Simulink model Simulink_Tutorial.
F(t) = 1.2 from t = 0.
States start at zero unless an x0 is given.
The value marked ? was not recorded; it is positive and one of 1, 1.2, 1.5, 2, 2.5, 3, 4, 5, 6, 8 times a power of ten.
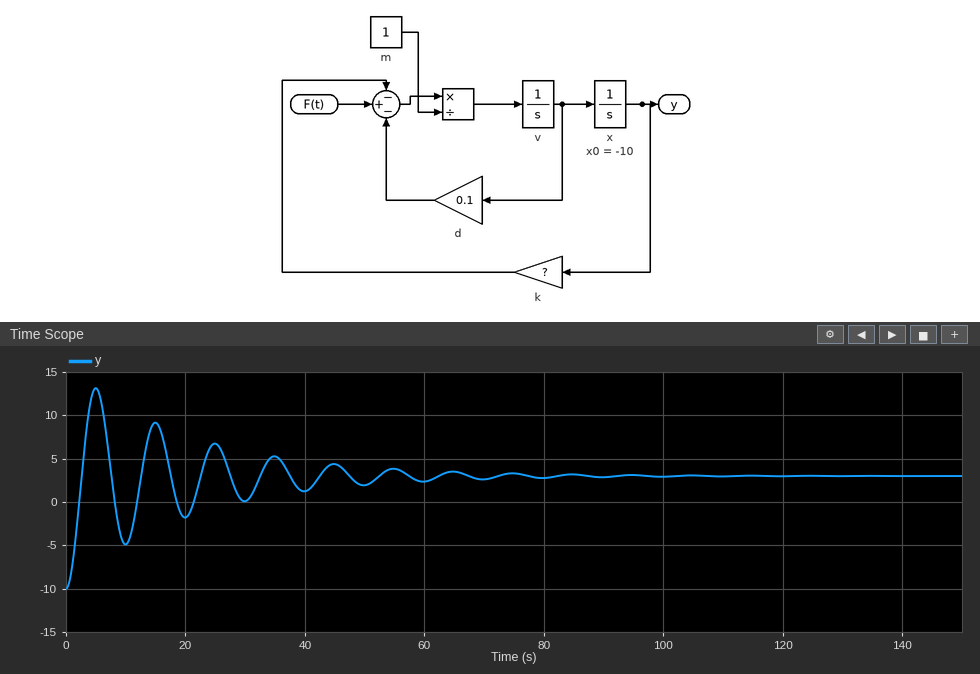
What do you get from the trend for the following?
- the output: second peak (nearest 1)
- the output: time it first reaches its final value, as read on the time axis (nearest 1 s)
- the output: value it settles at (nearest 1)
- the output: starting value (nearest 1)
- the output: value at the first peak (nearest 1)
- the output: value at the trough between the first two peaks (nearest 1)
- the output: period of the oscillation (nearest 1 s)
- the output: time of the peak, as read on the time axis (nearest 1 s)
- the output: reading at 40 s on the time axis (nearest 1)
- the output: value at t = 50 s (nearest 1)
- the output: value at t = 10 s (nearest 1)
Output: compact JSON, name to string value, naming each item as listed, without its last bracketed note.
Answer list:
{"the output: second peak": "9", "the output: time it first reaches its final value, as read on the time axis": "3 s", "the output: value it settles at": "3", "the output: starting value": "-10", "the output: value at the first peak": "13", "the output: value at the trough between the first two peaks": "-5", "the output: period of the oscillation": "10 s", "the output: time of the peak, as read on the time axis": "5 s", "the output: reading at 40 s on the time axis": "1", "the output: value at t = 50 s": "2", "the output: value at t = 10 s": "-5"}
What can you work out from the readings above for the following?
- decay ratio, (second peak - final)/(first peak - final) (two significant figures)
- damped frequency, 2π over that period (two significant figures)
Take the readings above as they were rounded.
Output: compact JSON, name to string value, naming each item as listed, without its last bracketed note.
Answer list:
{"decay ratio, (second peak - final)/(first peak - final)": "0.60", "damped frequency, 2π over that period": "0.63 rad/s"}
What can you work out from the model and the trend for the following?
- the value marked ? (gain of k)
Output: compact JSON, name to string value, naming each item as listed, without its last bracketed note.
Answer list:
{"the value marked ?": "0.4"}
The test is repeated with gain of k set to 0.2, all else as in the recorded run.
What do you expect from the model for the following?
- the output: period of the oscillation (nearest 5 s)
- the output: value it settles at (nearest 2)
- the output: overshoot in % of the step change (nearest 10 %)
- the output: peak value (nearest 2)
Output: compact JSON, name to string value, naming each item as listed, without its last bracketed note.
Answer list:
{"the output: period of the oscillation": "15 s", "the output: value it settles at": "6", "the output: overshoot in % of the step change": "70 %", "the output: peak value": "18"}
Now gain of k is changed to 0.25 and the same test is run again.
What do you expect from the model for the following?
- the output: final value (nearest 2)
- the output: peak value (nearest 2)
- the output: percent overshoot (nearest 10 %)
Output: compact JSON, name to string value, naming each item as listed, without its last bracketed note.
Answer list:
{"the output: final value": "4", "the output: peak value": "16", "the output: percent overshoot": "70 %"}
